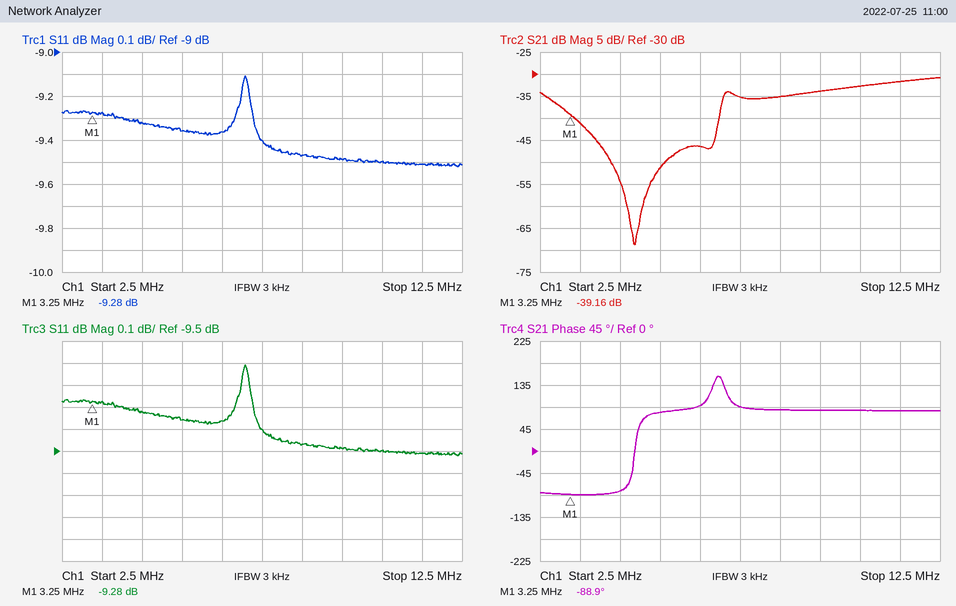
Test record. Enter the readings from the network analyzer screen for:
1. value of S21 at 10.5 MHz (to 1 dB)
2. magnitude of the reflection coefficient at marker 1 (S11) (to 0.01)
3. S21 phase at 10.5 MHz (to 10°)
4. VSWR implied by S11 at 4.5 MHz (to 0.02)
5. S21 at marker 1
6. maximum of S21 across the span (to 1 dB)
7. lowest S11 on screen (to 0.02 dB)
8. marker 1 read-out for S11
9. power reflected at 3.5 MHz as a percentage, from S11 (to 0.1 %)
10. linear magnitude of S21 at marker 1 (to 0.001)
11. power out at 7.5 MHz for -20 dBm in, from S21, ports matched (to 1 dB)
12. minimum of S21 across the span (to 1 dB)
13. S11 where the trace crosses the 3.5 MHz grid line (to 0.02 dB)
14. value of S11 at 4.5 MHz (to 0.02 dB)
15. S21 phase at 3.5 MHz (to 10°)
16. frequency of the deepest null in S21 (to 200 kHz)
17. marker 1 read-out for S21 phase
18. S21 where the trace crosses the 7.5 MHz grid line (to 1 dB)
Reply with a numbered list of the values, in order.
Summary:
1. -33 dB
2. 0.34
3. 80°
4. 2.04
5. -39.16 dB
6. -31 dB
7. -9.52 dB
8. -9.28 dB
9. 11.8 %
10. 0.011
11. -55 dBm
12. -69 dB
13. -9.28 dB
14. -9.32 dB
15. -90°
16. 4.8 MHz
17. -88.9°
18. -35 dB
